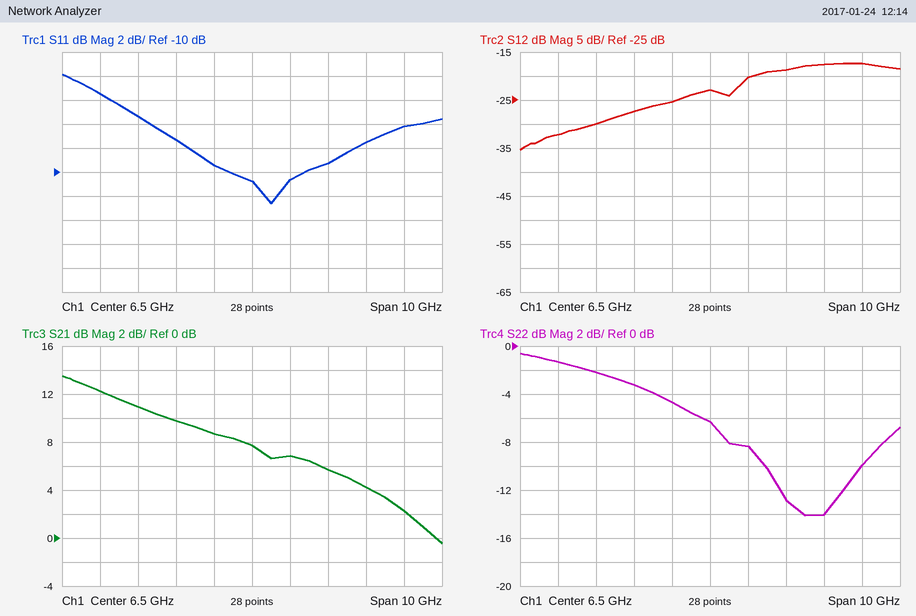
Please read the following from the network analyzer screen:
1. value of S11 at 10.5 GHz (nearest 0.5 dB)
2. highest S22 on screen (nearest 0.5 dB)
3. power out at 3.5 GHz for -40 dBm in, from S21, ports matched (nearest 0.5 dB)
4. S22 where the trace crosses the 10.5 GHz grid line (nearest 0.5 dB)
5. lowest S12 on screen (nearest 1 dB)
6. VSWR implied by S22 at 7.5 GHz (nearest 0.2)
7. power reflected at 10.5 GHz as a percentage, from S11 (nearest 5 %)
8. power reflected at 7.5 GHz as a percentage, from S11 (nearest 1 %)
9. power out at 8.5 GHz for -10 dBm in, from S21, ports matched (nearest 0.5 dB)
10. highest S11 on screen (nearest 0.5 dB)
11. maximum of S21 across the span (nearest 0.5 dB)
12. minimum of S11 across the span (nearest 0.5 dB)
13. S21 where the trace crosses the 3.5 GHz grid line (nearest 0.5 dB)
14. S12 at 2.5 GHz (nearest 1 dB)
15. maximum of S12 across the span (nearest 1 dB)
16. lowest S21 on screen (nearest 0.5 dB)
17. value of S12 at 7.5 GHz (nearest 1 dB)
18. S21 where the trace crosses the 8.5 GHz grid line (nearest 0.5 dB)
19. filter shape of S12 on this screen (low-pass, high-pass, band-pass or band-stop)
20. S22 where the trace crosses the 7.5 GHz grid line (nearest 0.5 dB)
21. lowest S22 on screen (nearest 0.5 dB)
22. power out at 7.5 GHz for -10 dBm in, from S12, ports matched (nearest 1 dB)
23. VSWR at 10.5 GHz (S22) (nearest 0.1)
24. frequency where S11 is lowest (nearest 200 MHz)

-6.0 dB
-0.5 dB
-29.0 dBm
-10.0 dB
-35 dB
2.2
25 %
9 %
-4.5 dBm
-2.0 dB
13.5 dB
-12.5 dB
11.0 dB
-32 dB
-17 dB
-0.5 dB
-20 dB
5.5 dB
high-pass
-8.5 dB
-14.0 dB
-30 dBm
1.9
7.0 GHz
